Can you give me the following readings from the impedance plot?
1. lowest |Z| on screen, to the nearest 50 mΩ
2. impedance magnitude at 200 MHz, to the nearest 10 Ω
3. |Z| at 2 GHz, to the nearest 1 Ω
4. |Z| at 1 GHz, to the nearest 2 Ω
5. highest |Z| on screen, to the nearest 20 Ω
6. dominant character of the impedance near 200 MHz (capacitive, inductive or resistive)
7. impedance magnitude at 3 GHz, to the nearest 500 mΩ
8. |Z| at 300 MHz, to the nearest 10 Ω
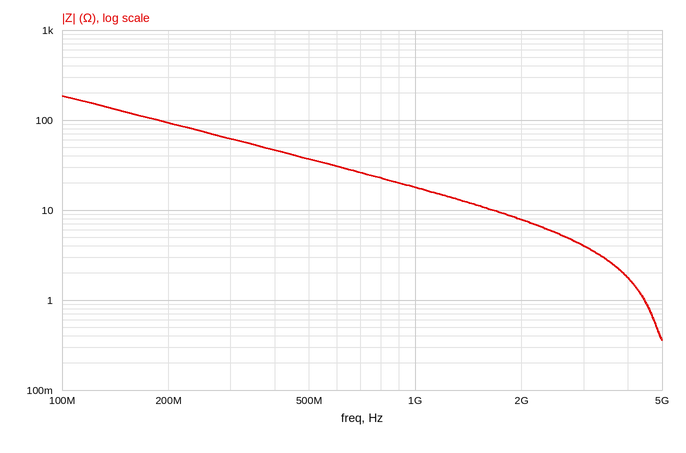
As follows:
350 mΩ
90 Ω
8 Ω
18 Ω
180 Ω
capacitive
4.0 Ω
60 Ω
